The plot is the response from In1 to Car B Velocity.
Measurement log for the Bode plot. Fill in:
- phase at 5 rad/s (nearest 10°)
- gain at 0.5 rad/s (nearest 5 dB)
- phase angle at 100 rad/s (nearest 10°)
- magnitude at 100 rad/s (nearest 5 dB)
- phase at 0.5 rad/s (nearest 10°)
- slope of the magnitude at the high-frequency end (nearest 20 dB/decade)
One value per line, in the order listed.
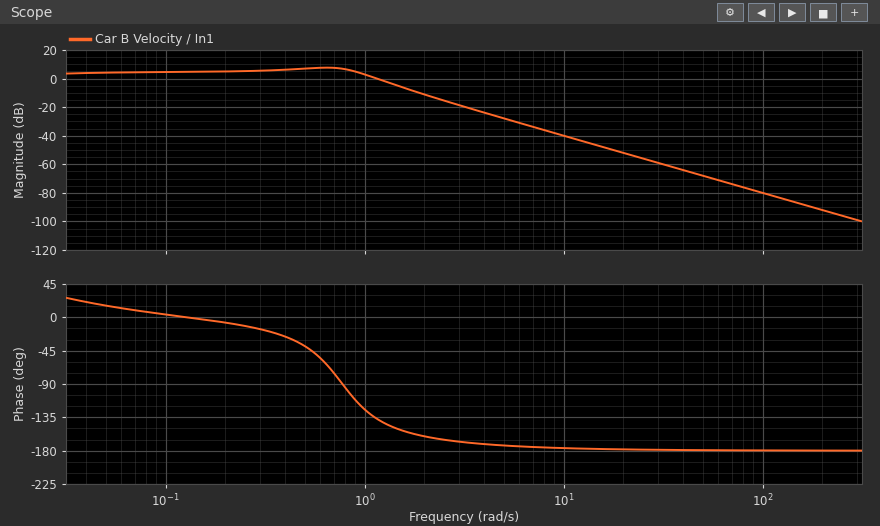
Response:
-170°
5 dB
-180°
-80 dB
-40°
-40 dB/decade
